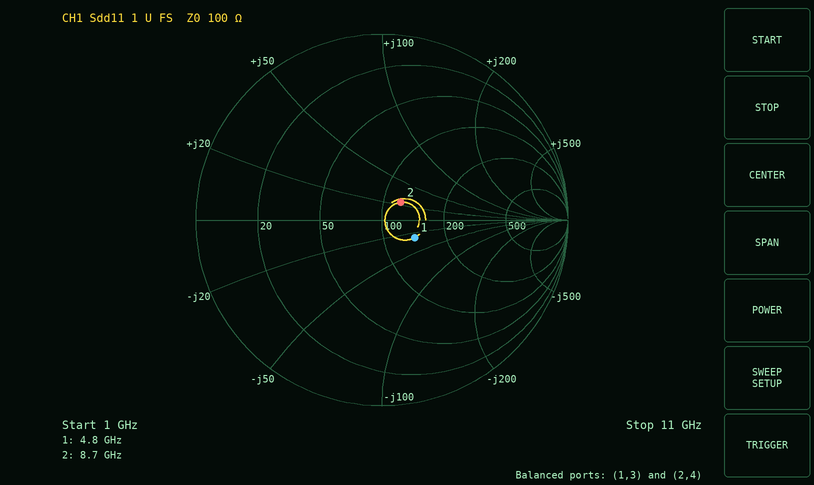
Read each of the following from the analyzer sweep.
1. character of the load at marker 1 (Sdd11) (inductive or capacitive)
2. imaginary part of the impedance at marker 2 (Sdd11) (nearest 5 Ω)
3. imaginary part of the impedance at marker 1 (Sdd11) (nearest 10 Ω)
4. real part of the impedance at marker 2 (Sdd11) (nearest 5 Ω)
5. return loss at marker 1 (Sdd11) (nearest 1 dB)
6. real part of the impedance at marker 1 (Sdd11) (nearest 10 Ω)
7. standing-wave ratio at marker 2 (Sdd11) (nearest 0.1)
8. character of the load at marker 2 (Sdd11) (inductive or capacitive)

capacitive
+25 Ω
-30 Ω
120 Ω
14 dB
140 Ω
1.3
inductive
